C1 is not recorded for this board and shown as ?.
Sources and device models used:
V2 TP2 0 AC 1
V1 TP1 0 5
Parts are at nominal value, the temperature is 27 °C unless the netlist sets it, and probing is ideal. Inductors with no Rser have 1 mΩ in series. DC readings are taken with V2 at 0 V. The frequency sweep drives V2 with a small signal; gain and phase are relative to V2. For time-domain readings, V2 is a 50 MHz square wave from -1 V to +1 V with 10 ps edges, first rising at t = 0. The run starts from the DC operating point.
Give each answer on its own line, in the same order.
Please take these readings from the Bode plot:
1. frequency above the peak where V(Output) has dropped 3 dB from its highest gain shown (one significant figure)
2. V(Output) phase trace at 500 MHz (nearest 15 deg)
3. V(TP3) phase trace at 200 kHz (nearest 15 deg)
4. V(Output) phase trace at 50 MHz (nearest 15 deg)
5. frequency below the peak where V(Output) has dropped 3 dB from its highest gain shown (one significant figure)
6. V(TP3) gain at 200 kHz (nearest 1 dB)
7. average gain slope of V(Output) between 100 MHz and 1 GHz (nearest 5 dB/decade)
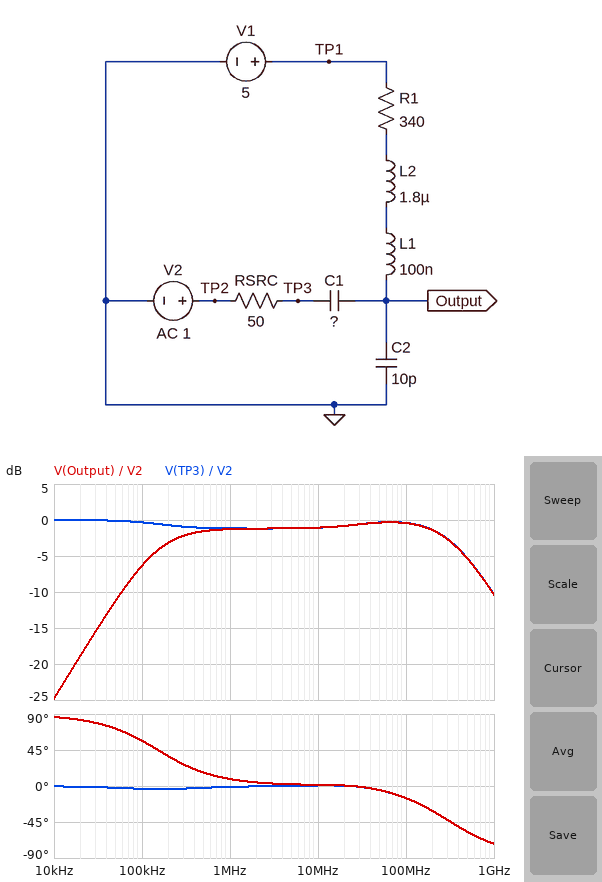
300 MHz
-60 deg
0 deg
0 deg
200 kHz
-1 dB
-10 dB/decade
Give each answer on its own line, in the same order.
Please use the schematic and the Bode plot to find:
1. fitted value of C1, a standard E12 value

2.7 nF
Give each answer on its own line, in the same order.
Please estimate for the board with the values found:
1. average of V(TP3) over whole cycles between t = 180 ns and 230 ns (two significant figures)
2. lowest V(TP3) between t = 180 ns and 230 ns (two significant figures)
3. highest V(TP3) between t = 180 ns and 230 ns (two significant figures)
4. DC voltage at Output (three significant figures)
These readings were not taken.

-110 mV
-1.1 V
920 mV
5.00 V
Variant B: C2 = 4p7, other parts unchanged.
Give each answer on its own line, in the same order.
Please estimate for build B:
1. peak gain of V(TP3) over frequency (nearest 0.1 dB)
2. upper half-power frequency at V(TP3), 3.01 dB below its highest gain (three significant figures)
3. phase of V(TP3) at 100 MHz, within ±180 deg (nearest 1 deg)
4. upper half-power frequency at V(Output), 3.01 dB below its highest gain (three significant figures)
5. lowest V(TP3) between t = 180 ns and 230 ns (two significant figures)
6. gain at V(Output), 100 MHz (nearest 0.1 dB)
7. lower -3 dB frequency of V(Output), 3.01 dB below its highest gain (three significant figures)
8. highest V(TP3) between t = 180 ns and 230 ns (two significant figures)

0 dB
682 MHz
-6 deg
704 MHz
-1.2 V
-0.2 dB
198 kHz
950 mV
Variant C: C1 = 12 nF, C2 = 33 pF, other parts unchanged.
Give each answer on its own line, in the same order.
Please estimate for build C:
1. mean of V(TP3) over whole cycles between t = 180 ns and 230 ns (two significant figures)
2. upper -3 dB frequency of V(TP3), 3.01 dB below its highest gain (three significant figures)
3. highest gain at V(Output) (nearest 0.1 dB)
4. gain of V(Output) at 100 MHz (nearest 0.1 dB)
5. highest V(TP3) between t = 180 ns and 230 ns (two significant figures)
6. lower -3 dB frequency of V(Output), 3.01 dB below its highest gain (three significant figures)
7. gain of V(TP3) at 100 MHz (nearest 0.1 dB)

-120 mV
99.4 MHz
-0.8 dB
-3.1 dB
830 mV
37.3 kHz
-3.0 dB
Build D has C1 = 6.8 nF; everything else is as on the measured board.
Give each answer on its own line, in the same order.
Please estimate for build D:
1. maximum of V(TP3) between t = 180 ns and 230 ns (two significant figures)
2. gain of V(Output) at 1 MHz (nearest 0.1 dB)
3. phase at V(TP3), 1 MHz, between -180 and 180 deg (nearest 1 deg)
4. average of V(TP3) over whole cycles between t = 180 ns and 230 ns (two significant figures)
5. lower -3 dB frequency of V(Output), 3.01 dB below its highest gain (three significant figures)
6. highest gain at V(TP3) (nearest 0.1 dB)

910 mV
-1.2 dB
0 deg
-120 mV
75.5 kHz
0 dB
